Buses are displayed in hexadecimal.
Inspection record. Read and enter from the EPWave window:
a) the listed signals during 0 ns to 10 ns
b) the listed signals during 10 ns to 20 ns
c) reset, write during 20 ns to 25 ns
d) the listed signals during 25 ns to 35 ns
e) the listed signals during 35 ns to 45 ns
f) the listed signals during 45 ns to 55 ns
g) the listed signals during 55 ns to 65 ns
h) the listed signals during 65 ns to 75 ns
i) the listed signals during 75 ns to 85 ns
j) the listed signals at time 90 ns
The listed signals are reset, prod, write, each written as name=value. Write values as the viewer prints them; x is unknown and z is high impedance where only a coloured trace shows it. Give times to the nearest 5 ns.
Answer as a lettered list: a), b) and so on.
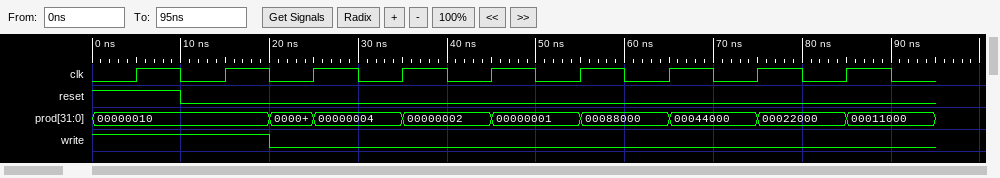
a) reset=1, prod=00000010, write=1
b) reset=0, prod=00000010, write=1
c) reset=0, write=0
d) reset=0, prod=00000004, write=0
e) reset=0, prod=00000002, write=0
f) reset=0, prod=00000001, write=0
g) reset=0, prod=00088000, write=0
h) reset=0, prod=00044000, write=0
i) reset=0, prod=00022000, write=0
j) reset=0, prod=00011000, write=0
